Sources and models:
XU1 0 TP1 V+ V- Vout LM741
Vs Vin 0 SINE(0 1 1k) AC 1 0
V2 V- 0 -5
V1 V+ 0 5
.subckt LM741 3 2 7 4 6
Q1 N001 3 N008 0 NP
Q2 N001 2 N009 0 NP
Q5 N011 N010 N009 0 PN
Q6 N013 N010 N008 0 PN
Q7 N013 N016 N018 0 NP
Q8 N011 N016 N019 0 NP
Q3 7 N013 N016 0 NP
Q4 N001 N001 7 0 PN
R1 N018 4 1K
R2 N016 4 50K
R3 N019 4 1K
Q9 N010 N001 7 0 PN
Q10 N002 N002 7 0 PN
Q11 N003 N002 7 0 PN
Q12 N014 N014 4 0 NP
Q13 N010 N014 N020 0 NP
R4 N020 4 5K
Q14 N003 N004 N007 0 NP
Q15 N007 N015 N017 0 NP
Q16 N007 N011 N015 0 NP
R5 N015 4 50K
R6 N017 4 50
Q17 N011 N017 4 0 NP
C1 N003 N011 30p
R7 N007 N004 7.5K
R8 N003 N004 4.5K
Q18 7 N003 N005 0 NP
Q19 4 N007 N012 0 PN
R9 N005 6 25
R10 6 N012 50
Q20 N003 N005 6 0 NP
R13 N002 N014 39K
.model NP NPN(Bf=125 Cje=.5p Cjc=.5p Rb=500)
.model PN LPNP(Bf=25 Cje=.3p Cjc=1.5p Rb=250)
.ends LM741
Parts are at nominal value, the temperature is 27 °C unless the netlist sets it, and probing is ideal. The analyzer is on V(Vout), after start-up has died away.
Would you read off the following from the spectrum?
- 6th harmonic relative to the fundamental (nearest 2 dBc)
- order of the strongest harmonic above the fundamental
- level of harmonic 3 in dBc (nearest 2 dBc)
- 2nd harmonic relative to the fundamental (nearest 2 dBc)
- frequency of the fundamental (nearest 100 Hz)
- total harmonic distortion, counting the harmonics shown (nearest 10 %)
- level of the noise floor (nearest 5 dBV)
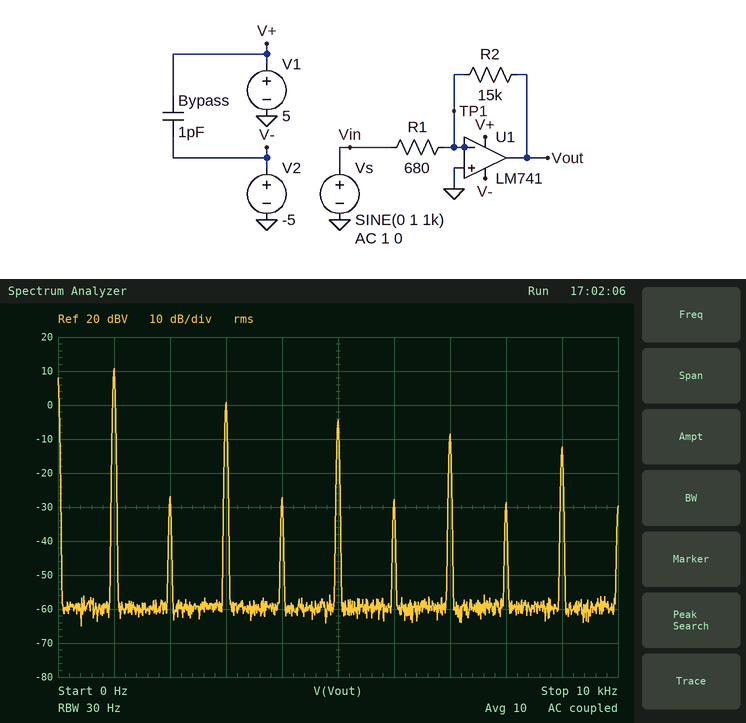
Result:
-38 dBc
3
-10 dBc
-38 dBc
1.0 kHz
40 %
-60 dBV
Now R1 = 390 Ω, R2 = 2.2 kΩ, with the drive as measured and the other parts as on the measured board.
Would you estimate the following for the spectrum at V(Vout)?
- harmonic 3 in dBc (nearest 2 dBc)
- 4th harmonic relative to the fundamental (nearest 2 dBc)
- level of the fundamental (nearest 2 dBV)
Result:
-16 dBc
-42 dBc
10 dBV
